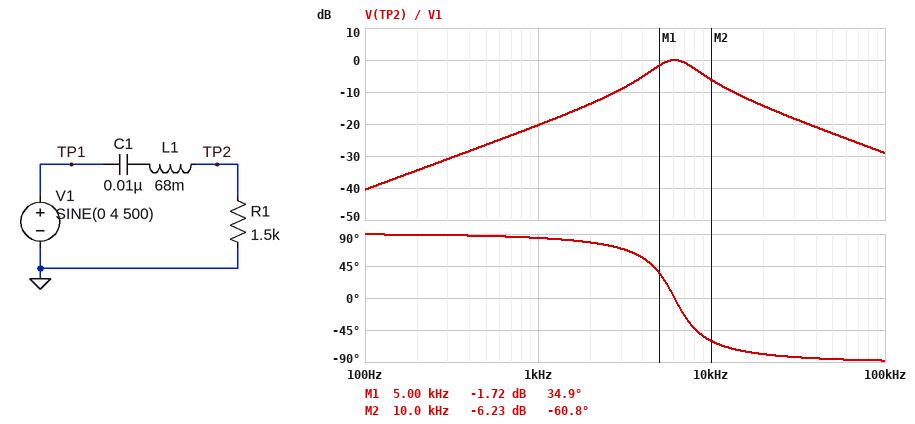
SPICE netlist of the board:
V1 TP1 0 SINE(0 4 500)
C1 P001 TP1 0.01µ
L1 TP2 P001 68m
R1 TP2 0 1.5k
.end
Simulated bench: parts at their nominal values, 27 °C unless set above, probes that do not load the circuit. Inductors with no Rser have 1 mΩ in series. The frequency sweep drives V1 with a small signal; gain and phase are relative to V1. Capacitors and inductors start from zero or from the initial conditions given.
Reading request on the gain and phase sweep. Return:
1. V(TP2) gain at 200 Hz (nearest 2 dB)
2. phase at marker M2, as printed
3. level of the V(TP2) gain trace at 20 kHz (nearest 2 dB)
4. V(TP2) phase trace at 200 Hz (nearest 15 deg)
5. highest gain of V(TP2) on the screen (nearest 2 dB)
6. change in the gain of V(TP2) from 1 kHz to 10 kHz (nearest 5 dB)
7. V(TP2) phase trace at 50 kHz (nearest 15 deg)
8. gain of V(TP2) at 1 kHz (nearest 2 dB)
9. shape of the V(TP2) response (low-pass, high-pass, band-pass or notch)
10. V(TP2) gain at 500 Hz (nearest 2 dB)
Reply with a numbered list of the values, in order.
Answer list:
1. -34 dB
2. -60.8 deg
3. -14 dB
4. 90 deg
5. 0 dB
6. 15 dB
7. -90 deg
8. -20 dB
9. band-pass
10. -26 dB
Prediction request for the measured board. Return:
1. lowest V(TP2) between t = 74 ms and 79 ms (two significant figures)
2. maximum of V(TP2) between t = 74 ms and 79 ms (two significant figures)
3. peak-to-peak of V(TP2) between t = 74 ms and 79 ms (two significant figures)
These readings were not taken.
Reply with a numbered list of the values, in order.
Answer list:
1. -190 mV
2. 190 mV
3. 380 mV
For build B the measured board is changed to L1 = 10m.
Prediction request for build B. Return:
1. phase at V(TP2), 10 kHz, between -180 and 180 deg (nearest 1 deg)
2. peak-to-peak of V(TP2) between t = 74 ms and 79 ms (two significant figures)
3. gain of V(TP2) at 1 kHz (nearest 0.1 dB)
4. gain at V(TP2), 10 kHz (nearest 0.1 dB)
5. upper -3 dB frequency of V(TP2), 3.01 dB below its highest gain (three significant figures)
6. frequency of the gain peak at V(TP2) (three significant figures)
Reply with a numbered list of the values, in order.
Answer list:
1. 33 deg
2. 380 mV
3. -20.5 dB
4. -1.5 dB
5. 31.8 kHz
6. 15.9 kHz
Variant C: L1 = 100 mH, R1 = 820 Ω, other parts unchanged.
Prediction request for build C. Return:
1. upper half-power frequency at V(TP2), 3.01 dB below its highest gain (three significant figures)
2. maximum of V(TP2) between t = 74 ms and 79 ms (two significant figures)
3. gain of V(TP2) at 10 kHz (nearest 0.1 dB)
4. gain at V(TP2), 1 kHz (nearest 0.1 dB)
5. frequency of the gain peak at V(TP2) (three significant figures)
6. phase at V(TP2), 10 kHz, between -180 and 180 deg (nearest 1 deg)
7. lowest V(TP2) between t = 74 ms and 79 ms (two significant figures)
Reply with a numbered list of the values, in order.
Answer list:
1. 5.73 kHz
2. 100 mV
3. -15.3 dB
4. -25.4 dB
5. 5.03 kHz
6. -80 deg
7. -100 mV
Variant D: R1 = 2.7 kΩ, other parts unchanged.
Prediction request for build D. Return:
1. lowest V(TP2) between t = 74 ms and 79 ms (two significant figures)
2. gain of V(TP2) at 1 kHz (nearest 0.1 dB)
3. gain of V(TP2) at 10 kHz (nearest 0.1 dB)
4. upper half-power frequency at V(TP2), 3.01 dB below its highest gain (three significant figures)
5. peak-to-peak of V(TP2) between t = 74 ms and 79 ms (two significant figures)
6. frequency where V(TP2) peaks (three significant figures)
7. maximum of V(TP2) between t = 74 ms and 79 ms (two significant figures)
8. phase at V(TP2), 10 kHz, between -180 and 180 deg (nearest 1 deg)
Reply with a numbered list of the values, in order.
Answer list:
1. -340 mV
2. -15.3 dB
3. -3.0 dB
4. 10.0 kHz
5. 680 mV
6. 6.10 kHz
7. 340 mV
8. -45 deg
